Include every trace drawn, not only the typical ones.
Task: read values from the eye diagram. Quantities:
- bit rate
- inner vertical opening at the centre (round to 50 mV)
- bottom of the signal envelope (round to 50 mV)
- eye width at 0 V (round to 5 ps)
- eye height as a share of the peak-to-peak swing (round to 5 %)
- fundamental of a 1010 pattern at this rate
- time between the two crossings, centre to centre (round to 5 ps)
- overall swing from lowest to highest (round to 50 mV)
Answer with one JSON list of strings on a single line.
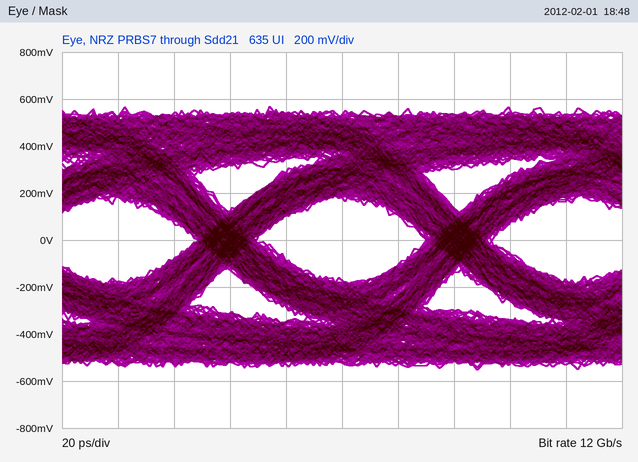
["12 Gb/s", "350 mV", "-550 mV", "60 ps", "30 %", "6 GHz", "85 ps", "1.10 V"]
